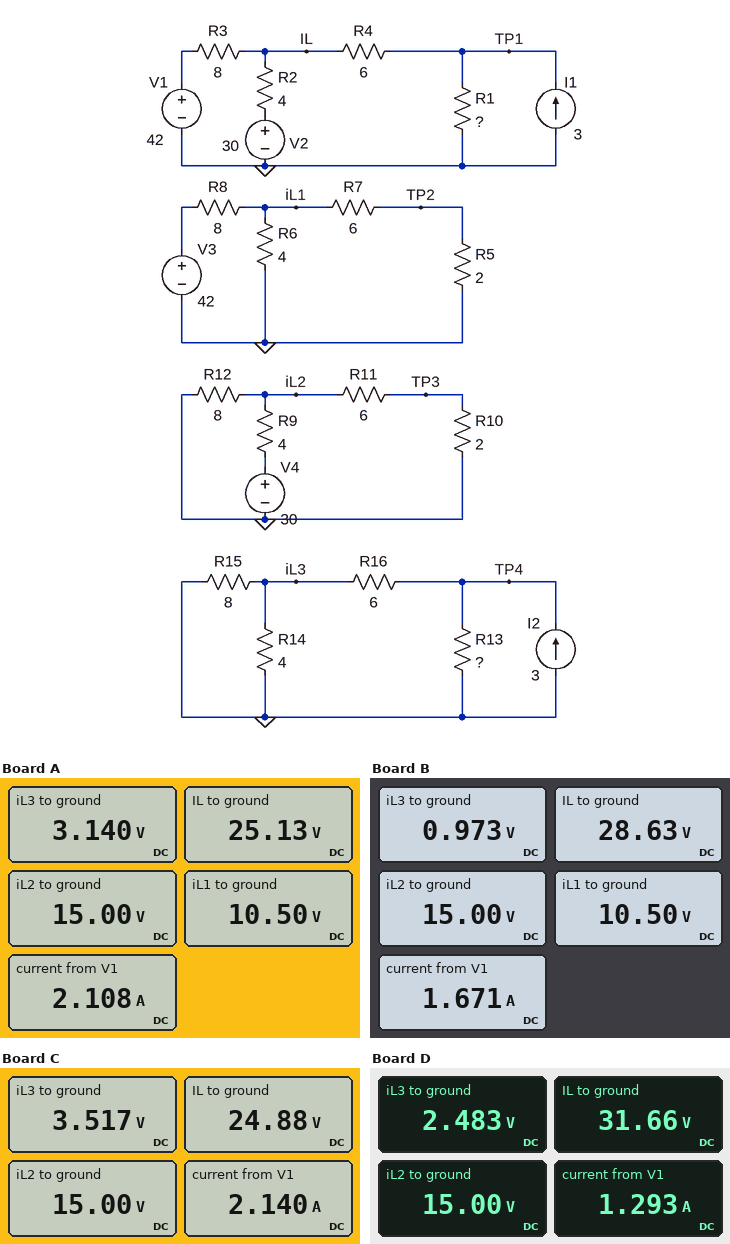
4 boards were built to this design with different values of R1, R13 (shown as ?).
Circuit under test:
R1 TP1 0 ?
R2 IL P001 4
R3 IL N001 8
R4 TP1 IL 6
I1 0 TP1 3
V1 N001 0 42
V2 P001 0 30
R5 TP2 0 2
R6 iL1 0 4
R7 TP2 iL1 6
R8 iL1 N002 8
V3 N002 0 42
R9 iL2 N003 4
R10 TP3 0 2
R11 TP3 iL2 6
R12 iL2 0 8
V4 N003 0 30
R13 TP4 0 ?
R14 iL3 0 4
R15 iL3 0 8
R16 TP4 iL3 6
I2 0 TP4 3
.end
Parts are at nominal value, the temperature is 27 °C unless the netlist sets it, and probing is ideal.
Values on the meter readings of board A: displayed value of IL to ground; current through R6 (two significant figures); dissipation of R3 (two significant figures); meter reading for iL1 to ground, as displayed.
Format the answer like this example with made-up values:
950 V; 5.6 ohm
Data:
25.13 V; 2.6 A; 36 W; 10.50 V
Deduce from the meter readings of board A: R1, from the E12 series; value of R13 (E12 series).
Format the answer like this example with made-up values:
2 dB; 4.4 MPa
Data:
0.82 Ω; 5.6 Ω
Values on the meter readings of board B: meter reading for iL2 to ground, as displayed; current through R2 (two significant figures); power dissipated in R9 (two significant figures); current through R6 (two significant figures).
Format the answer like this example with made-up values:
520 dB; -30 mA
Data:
15.00 V; 340 mA; 56 W; 2.6 A
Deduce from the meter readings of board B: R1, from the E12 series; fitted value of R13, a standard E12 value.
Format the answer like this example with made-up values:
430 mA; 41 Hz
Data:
3.3 Ω; 1.2 Ω
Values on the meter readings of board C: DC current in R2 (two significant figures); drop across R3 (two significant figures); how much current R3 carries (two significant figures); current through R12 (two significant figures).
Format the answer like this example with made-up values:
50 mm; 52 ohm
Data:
1.3 A; 17 V; 2.1 A; 1.9 A
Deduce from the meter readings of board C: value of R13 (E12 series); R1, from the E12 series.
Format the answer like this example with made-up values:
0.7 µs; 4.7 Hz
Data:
6.8 Ω; 0.68 Ω
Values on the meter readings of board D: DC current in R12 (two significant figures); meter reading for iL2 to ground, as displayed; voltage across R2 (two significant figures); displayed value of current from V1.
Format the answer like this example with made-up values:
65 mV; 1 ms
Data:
1.9 A; 15.00 V; 1.7 V; 1.293 A
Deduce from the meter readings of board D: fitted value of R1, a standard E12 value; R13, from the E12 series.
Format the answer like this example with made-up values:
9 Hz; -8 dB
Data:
6.8 Ω; 3.9 Ω
